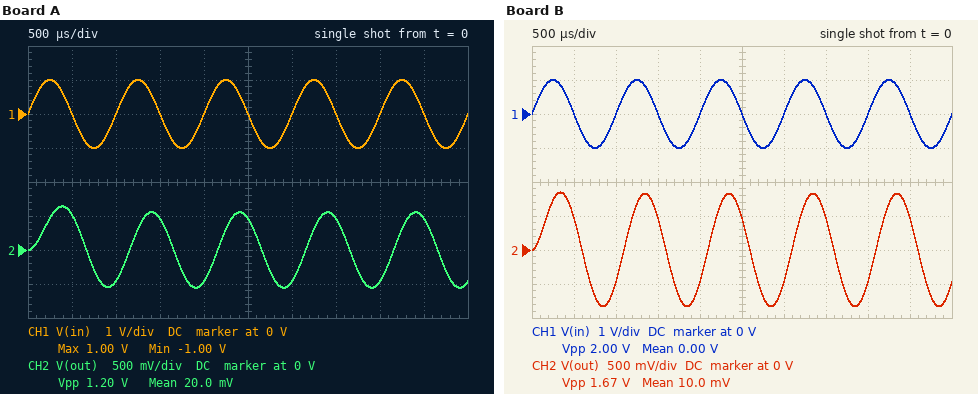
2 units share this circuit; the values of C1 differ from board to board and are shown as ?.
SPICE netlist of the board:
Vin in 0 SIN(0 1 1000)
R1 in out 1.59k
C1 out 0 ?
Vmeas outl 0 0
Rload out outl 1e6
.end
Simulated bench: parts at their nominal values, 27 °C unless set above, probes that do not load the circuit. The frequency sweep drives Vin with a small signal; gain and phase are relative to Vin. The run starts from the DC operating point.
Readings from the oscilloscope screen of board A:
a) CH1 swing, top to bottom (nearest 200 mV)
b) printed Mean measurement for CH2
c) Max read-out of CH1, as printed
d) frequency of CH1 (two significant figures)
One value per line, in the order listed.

2.0 V
20.0 mV
1.00 V
1.0 kHz
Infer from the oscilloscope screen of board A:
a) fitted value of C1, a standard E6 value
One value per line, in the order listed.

150 nF
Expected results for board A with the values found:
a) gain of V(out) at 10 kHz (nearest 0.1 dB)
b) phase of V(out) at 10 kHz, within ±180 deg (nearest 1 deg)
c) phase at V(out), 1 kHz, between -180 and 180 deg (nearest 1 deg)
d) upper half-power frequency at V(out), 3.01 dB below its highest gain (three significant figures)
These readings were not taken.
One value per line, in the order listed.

-23.5 dB
-86 deg
-56 deg
668 Hz
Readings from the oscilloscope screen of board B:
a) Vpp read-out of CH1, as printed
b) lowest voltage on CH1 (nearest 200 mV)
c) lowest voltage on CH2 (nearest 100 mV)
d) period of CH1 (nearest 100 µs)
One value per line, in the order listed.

2.00 V
-1.0 V
-800 mV
1.0 ms
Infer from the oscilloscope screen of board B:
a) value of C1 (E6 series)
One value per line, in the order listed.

68 nF
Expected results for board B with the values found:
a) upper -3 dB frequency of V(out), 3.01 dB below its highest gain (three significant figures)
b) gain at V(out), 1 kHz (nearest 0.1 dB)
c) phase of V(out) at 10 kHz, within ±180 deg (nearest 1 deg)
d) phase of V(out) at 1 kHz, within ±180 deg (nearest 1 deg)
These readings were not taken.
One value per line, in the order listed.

1.47 kHz
-1.7 dB
-82 deg
-34 deg
